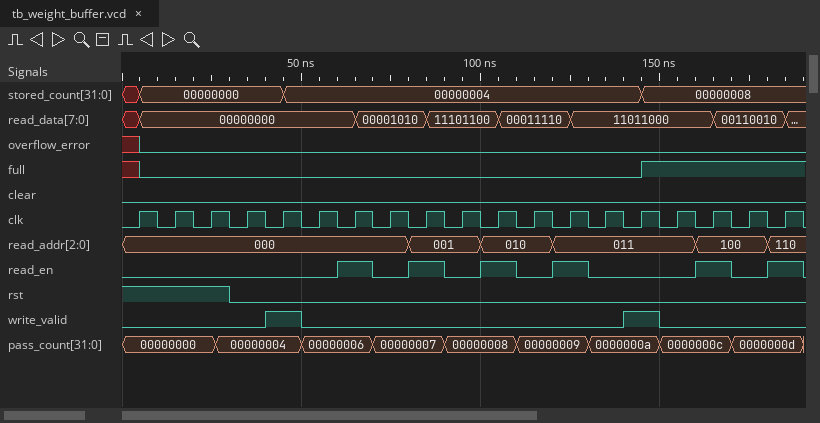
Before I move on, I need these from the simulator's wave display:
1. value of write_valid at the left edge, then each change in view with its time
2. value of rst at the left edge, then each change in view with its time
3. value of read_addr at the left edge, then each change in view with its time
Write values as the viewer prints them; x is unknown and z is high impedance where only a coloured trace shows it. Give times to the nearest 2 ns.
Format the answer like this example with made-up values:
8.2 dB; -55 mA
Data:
0, 1 at 40 ns, 0 at 50 ns, 1 at 140 ns, 0 at 150 ns; 1, 0 at 30 ns; 000, 001 at 80 ns, 010 at 100 ns, 011 at 120 ns, 100 at 160 ns, 110 at 180 ns
